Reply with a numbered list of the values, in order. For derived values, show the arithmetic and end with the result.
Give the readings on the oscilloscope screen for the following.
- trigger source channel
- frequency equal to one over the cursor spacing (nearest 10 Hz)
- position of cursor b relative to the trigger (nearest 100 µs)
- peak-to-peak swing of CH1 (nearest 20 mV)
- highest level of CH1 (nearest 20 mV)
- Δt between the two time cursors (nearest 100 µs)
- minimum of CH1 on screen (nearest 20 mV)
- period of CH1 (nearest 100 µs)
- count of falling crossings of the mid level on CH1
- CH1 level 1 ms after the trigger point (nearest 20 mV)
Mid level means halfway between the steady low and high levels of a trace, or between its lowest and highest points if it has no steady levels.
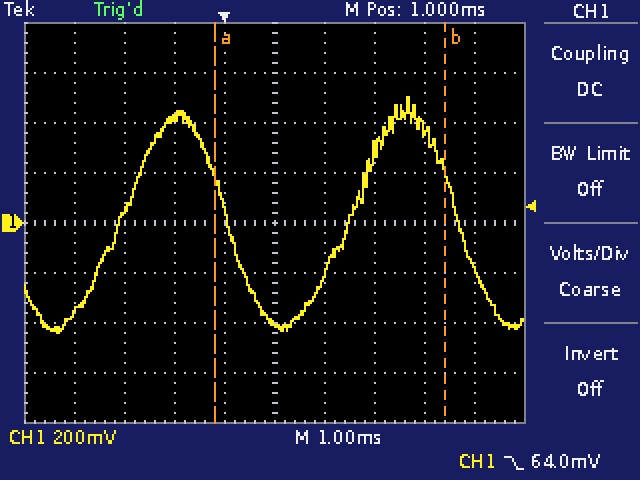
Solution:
1. CH1
2. 1 / 4.6 ms ≈ 220 Hz
3. +4.4 ms
4. 500 mV − (-440 mV) = 940 mV
5. 500 mV
6. 4.6 ms
7. -440 mV
8. 4.6 ms
9. 2
10. -400 mV
